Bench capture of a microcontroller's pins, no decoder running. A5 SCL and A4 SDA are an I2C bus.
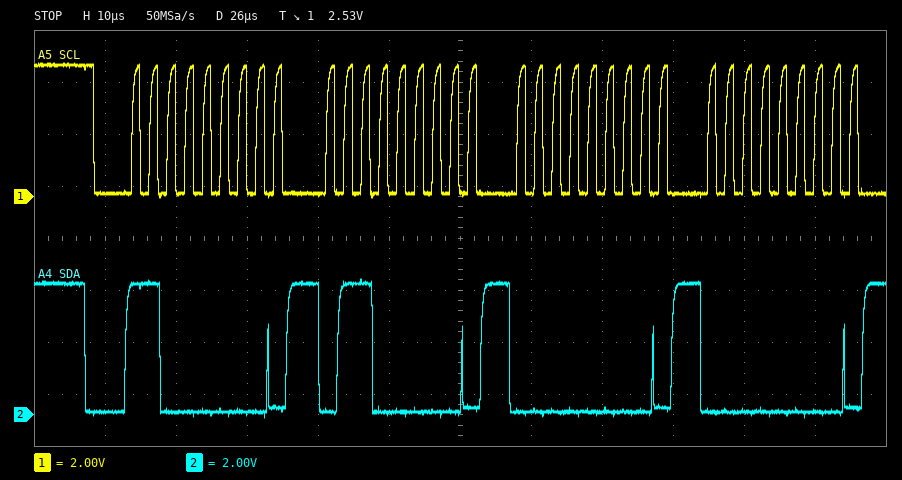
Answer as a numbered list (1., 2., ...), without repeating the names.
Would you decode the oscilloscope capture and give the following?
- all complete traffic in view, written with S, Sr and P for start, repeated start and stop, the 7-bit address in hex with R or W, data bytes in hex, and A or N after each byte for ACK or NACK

1. S 60W A 60 A 00 A 00 A
